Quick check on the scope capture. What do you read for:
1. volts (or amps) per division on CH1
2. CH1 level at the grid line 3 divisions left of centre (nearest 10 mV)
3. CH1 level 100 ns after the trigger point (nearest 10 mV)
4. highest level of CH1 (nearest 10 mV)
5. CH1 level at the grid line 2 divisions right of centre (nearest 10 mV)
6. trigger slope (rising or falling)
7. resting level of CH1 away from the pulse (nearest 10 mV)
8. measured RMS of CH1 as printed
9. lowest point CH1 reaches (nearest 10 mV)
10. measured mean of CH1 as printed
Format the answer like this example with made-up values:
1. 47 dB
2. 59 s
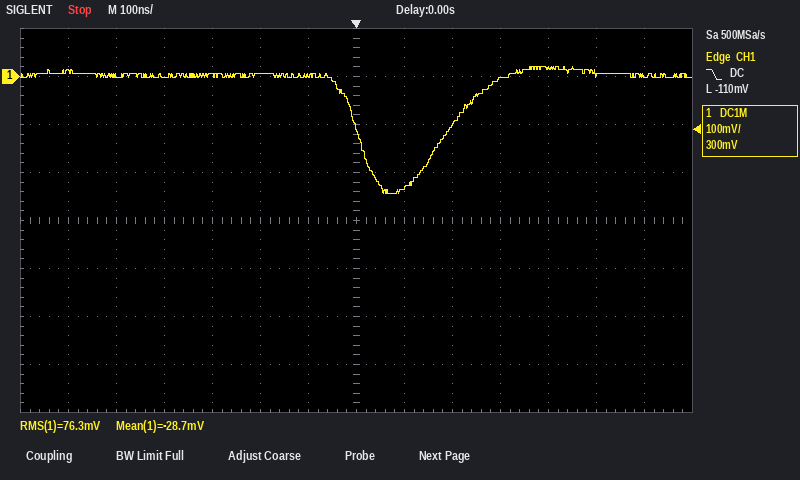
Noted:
1. 100 mV
2. 0 mV
3. -230 mV
4. 20 mV
5. -100 mV
6. falling
7. 0 mV
8. 76.3 mV
9. -240 mV
10. -28.7 mV
